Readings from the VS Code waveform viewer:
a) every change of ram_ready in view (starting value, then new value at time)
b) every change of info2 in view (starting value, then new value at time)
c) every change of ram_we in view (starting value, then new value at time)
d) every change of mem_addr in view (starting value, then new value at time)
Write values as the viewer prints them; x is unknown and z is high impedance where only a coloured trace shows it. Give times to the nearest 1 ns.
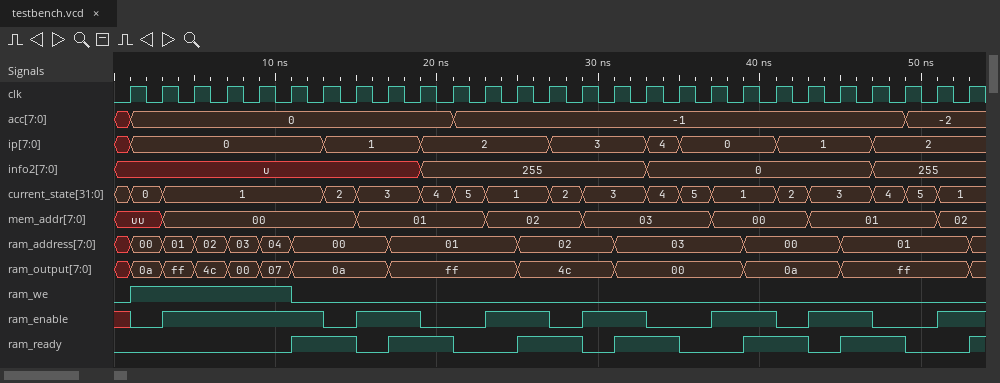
0, 1 at 11 ns, 0 at 15 ns, 1 at 17 ns, 0 at 21 ns, 1 at 25 ns, 0 at 29 ns, 1 at 31 ns, 0 at 35 ns, 1 at 39 ns, 0 at 43 ns, 1 at 45 ns, 0 at 49 ns, 1 at 53 ns
u, 255 at 19 ns, 0 at 33 ns, 255 at 47 ns
0, 1 at 1 ns, 0 at 11 ns
uu, 00 at 3 ns, 01 at 15 ns, 02 at 23 ns, 03 at 29 ns, 00 at 37 ns, 01 at 43 ns, 02 at 51 ns
